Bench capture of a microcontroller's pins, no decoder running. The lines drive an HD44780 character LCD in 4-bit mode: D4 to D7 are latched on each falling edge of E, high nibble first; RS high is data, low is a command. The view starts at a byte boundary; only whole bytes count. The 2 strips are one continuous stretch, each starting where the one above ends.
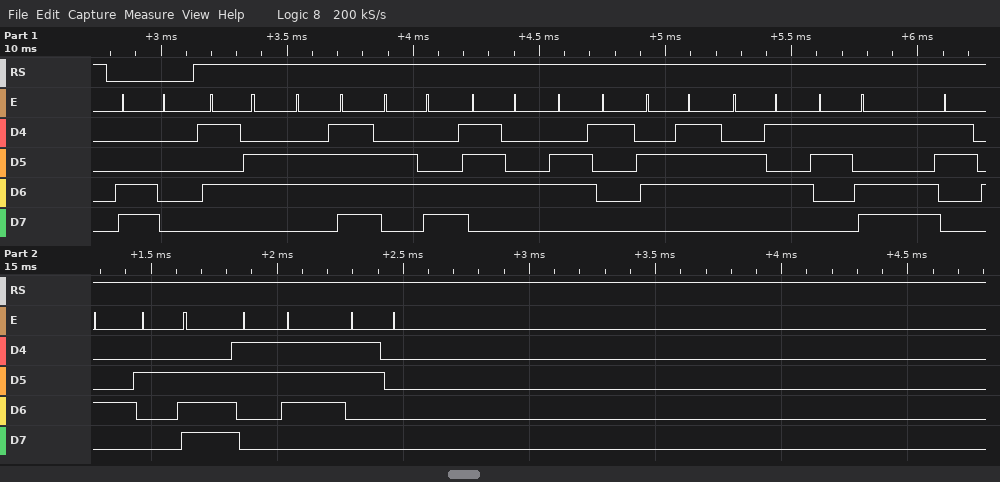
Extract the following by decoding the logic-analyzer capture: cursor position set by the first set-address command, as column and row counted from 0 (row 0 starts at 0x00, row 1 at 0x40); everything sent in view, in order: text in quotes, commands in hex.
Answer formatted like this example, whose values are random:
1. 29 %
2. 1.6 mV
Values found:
1. column 0, row 1
2. 0xC0 "Voltage=4.70"
